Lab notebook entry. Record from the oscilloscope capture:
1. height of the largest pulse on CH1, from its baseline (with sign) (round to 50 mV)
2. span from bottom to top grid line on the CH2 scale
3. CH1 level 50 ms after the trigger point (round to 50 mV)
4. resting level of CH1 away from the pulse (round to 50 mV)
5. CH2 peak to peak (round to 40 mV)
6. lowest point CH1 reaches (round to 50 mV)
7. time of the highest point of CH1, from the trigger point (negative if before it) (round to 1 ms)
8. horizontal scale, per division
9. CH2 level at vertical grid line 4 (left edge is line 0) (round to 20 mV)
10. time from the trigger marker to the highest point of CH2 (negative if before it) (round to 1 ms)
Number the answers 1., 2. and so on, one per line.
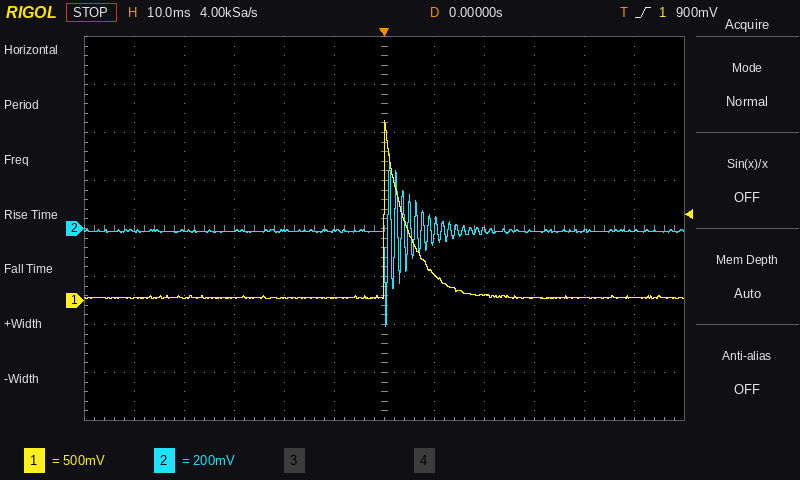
1. +1.85 V
2. 1.6 V
3. 50 mV
4. 50 mV
5. 720 mV
6. 0 mV
7. 0 ms
8. 10 ms
9. 0 mV
10. +1 ms
